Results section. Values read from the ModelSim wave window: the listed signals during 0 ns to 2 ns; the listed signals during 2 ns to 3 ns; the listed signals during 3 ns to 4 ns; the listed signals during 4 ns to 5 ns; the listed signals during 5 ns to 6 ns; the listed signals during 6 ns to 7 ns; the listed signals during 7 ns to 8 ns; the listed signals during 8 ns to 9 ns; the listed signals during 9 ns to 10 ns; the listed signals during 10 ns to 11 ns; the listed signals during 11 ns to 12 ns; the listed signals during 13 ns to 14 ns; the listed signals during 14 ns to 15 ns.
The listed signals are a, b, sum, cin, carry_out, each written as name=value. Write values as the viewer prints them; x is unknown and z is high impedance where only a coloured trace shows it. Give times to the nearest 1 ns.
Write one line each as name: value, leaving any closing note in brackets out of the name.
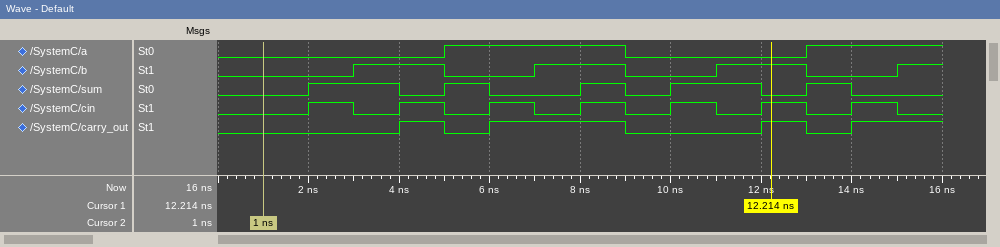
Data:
the listed signals during 0 ns to 2 ns: a=0, b=0, sum=0, cin=0, carry_out=0
the listed signals during 2 ns to 3 ns: a=0, b=0, sum=1, cin=1, carry_out=0
the listed signals during 3 ns to 4 ns: a=0, b=1, sum=1, cin=0, carry_out=0
the listed signals during 4 ns to 5 ns: a=0, b=1, sum=0, cin=1, carry_out=1
the listed signals during 5 ns to 6 ns: a=1, b=0, sum=1, cin=0, carry_out=0
the listed signals during 6 ns to 7 ns: a=1, b=0, sum=0, cin=1, carry_out=1
the listed signals during 7 ns to 8 ns: a=1, b=1, sum=0, cin=0, carry_out=1
the listed signals during 8 ns to 9 ns: a=1, b=1, sum=1, cin=1, carry_out=1
the listed signals during 9 ns to 10 ns: a=0, b=0, sum=0, cin=0, carry_out=0
the listed signals during 10 ns to 11 ns: a=0, b=0, sum=1, cin=1, carry_out=0
the listed signals during 11 ns to 12 ns: a=0, b=1, sum=1, cin=0, carry_out=0
the listed signals during 13 ns to 14 ns: a=1, b=0, sum=1, cin=0, carry_out=0
the listed signals during 14 ns to 15 ns: a=1, b=0, sum=0, cin=1, carry_out=1
